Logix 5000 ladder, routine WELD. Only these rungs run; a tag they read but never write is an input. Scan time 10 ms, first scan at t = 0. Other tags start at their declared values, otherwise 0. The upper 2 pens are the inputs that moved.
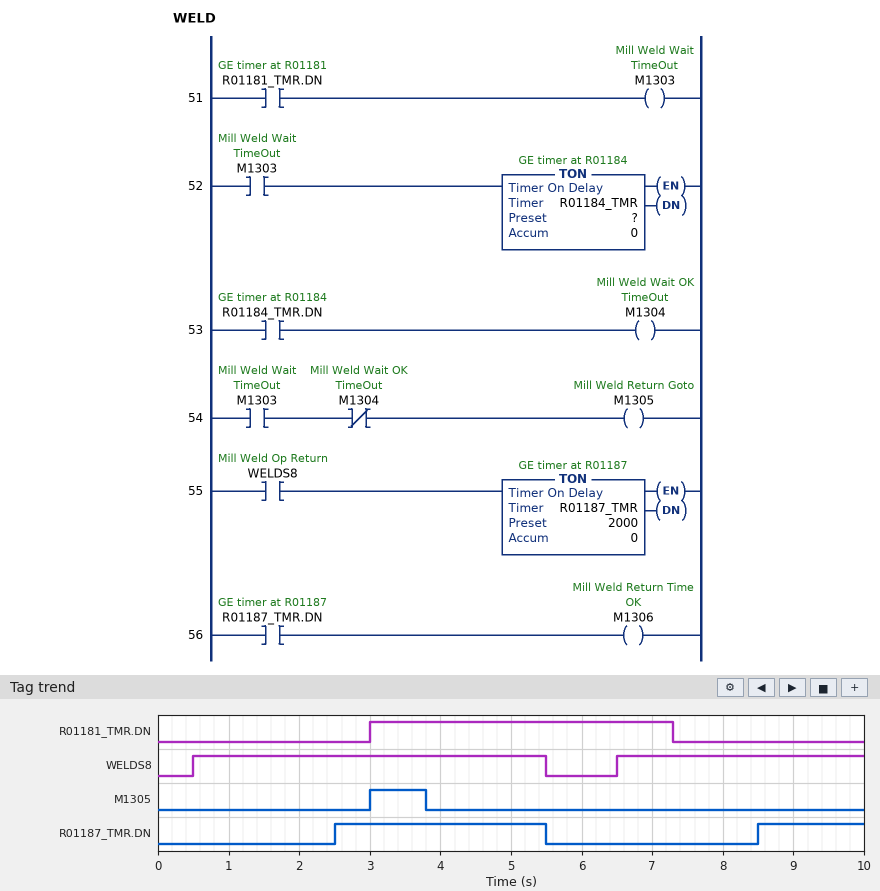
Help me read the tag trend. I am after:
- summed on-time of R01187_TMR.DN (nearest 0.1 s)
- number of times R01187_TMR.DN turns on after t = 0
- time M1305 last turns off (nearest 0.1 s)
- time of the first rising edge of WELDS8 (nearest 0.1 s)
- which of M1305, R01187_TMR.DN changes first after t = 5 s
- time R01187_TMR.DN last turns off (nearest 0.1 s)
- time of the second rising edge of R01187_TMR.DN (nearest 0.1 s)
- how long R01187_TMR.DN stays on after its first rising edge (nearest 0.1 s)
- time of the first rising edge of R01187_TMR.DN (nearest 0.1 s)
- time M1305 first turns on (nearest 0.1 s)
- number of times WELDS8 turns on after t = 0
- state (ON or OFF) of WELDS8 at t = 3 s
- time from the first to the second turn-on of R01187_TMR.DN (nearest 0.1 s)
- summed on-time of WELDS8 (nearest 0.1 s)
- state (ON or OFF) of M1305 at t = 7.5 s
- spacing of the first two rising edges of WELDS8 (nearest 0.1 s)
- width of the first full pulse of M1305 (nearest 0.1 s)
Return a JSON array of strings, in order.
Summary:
["4.5 s", "2", "3.8 s", "0.5 s", "R01187_TMR.DN", "5.5 s", "8.5 s", "3.0 s", "2.5 s", "3.0 s", "2", "ON", "6.0 s", "8.5 s", "OFF", "6.0 s", "0.8 s"]
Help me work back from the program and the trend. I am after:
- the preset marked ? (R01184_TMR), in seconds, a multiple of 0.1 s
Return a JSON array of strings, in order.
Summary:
["0.8 s"]
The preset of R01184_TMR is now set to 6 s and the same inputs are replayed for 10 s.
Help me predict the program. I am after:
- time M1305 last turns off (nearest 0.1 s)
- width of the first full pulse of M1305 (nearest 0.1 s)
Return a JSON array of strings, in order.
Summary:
["7.3 s", "4.3 s"]
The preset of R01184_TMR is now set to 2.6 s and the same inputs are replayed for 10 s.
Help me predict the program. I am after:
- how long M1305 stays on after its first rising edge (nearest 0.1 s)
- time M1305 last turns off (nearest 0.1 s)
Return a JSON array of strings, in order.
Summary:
["2.6 s", "5.6 s"]
